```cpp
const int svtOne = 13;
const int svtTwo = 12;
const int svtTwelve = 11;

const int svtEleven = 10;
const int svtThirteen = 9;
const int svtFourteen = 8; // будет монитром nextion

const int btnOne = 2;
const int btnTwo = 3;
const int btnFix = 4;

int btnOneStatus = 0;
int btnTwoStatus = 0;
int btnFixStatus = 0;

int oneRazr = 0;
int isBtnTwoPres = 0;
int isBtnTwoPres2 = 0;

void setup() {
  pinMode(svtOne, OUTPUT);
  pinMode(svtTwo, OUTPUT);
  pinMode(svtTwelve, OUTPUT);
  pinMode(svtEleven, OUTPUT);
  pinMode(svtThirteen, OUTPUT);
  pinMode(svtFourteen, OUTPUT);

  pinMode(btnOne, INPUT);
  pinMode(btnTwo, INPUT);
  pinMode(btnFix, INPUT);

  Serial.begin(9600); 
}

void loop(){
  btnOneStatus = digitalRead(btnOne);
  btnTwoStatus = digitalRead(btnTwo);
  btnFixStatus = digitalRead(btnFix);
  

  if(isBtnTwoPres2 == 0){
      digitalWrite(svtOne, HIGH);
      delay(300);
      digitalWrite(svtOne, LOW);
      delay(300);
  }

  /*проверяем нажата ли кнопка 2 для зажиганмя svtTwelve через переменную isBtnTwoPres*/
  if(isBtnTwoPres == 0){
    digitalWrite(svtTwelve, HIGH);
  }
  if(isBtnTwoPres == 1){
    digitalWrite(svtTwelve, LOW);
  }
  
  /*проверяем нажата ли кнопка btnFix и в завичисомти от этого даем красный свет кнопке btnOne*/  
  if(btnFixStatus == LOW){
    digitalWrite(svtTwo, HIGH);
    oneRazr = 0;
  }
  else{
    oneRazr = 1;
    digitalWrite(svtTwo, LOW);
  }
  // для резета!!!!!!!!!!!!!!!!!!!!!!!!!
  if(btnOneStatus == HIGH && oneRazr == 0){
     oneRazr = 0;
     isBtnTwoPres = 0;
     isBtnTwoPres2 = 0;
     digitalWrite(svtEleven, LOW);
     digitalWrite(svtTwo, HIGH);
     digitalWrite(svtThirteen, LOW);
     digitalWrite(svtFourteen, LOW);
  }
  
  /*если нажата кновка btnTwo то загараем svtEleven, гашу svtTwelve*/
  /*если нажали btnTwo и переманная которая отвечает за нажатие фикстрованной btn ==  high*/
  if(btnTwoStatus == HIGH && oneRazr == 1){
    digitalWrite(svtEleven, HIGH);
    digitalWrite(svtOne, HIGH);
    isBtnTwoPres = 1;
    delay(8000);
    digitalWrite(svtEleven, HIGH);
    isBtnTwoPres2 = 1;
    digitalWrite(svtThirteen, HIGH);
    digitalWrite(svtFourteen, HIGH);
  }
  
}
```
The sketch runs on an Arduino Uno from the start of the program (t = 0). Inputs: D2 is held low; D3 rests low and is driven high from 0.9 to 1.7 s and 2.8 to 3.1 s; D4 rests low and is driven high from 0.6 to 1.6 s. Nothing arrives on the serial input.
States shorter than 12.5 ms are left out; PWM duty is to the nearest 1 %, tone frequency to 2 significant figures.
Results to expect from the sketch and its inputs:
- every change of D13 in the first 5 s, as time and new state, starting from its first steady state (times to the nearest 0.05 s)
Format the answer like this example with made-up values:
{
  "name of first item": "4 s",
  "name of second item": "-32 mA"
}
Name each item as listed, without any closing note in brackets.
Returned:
{
  "every change of D13 in the first 5 s, as time and new state, starting from its first steady state": "0 s high; 0.3 s low; 0.6 s high; 0.9 s low; 1.2 s high; 1.5 s low; 1.8 s high"
}
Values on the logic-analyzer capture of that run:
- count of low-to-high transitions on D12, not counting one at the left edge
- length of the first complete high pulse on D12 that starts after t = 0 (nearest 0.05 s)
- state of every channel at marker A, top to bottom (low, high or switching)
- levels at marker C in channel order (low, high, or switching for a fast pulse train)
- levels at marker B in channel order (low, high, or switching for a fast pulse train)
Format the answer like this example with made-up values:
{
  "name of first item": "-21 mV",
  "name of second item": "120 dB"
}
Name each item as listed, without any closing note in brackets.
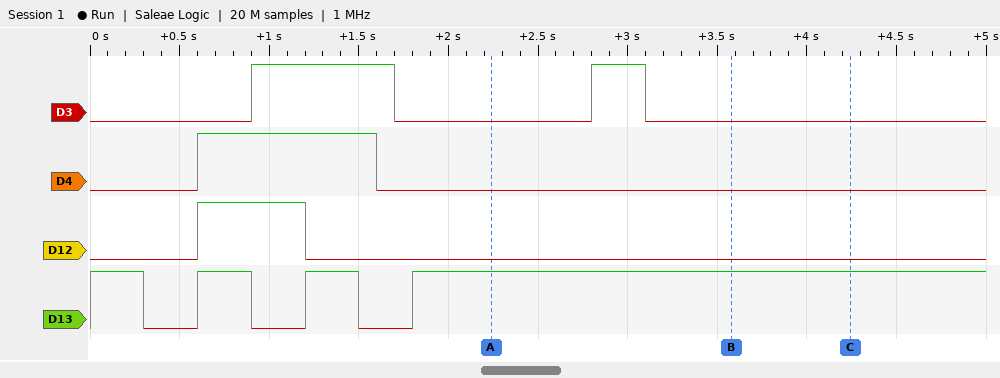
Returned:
{
  "count of low-to-high transitions on D12, not counting one at the left edge": "1",
  "length of the first complete high pulse on D12 that starts after t = 0": "0.60 s",
  "state of every channel at marker A, top to bottom": "D3 low, D4 low, D12 low, D13 high",
  "levels at marker C in channel order": "D3 low, D4 low, D12 low, D13 high",
  "levels at marker B in channel order": "D3 low, D4 low, D12 low, D13 high"
}
